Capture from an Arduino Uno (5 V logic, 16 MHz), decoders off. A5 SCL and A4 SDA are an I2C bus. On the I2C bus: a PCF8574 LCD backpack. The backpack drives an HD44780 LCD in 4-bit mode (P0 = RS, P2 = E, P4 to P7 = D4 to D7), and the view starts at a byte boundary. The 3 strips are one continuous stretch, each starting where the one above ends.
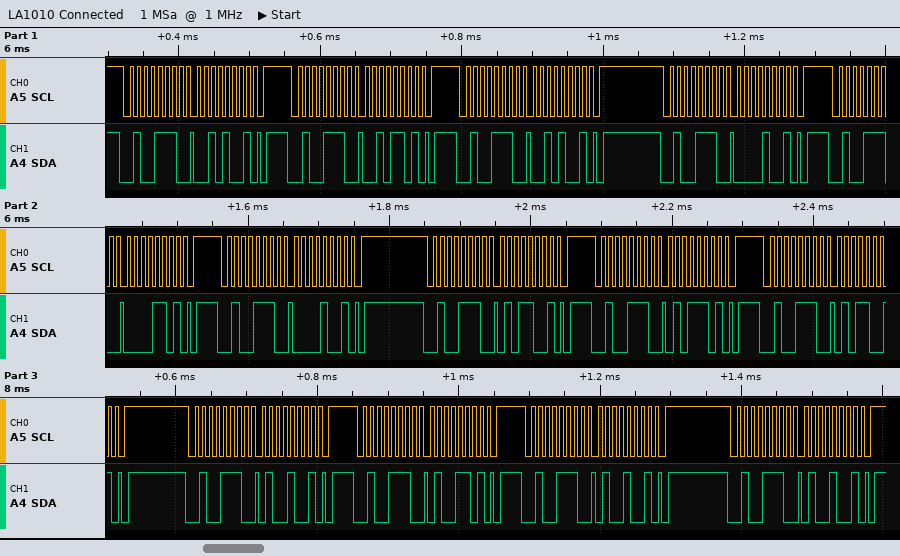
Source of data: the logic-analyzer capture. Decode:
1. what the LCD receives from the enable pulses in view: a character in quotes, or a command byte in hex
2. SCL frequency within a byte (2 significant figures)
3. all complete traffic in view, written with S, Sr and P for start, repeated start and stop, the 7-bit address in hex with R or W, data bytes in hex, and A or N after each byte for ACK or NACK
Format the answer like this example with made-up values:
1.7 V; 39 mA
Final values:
' ' 'T'; 100 kHz; S 27W A 29 A P S 27W A 2D A P S 27W A 29 A P S 27W A 09 A P S 27W A 0D A P S 27W A 09 A P S 27W A 59 A P S 27W A 5D A P S 27W A 59 A P S 27W A 49 A P S 27W A 4D A P S 27W A 49 A P S 27W A 49 A P
